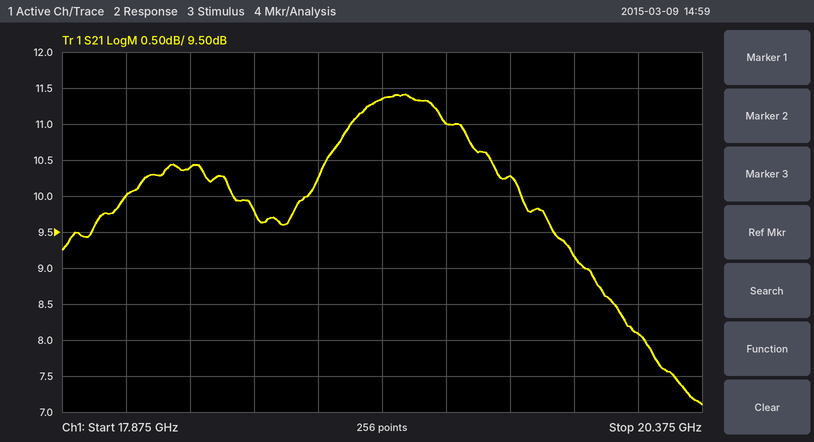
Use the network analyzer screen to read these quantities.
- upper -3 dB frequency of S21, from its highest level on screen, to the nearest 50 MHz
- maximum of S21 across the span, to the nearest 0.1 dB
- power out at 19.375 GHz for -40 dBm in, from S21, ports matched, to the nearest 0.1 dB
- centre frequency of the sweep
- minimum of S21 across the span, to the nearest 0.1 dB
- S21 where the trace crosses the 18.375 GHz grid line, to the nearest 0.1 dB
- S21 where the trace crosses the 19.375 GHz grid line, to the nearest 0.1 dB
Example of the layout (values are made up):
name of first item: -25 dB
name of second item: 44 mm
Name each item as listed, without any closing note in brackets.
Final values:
upper -3 dB frequency of S21, from its highest level on screen, to the nearest 50 MHz: 20.05 GHz
maximum of S21 across the span, to the nearest 0.1 dB: 11.4 dB
power out at 19.375 GHz for -40 dBm in, from S21, ports matched, to the nearest 0.1 dB: -29.0 dBm
centre frequency of the sweep: 19.125 GHz
minimum of S21 across the span, to the nearest 0.1 dB: 7.1 dB
S21 where the trace crosses the 18.375 GHz grid line, to the nearest 0.1 dB: 10.4 dB
S21 where the trace crosses the 19.375 GHz grid line, to the nearest 0.1 dB: 11.0 dB
